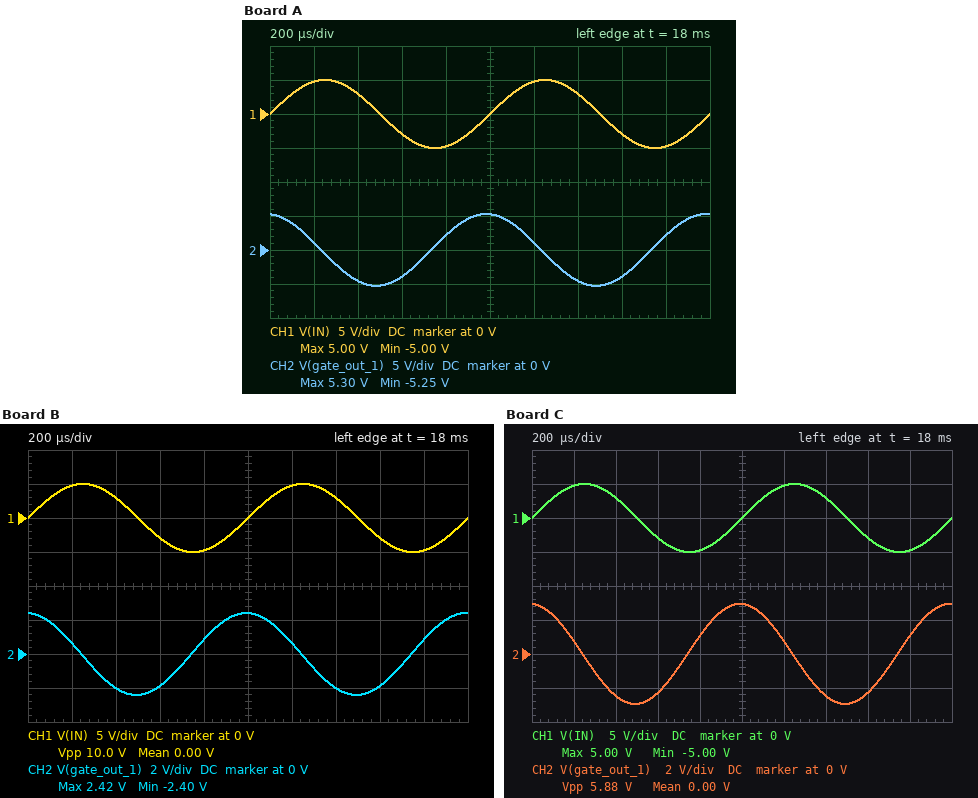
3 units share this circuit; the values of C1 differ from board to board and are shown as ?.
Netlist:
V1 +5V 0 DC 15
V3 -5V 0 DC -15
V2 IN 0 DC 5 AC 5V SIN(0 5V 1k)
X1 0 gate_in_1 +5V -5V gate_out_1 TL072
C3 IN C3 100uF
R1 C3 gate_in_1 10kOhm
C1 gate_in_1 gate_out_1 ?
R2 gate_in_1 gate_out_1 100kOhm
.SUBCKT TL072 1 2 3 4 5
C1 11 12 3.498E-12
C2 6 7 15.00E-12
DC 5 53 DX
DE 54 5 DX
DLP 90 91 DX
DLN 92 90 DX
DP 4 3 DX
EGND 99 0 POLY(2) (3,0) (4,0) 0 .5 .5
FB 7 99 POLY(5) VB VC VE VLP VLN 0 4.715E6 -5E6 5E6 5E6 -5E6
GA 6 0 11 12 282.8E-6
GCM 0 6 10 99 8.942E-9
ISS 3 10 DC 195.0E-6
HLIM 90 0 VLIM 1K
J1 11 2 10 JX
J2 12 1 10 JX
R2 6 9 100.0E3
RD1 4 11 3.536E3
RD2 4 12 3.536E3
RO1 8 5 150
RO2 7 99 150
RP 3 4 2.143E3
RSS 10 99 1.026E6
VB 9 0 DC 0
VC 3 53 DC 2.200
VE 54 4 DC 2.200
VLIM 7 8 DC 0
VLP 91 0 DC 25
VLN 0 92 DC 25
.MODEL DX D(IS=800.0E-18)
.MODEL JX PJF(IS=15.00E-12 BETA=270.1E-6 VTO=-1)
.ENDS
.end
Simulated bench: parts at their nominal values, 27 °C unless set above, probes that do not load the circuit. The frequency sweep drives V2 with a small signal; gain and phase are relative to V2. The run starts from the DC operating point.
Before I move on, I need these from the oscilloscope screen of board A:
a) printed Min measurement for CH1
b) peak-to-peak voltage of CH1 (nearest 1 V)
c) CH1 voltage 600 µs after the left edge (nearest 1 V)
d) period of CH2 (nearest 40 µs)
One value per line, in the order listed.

-5.00 V
10 V
-3 V
1.00 ms
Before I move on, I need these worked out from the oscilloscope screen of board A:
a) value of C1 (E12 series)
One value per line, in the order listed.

15 nF
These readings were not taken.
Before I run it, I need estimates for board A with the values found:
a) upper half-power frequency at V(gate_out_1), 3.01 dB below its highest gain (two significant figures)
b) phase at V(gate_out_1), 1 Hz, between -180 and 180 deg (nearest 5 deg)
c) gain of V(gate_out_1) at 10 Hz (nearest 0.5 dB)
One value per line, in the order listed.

110 Hz
-170 deg
20.0 dB
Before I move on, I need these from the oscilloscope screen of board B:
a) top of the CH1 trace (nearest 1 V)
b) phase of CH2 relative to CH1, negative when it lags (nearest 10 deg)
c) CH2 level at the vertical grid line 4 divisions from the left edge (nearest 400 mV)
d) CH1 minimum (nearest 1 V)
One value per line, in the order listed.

5 V
90 deg
800 mV
-5 V
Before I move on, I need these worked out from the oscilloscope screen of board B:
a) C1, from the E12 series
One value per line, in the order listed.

33 nF
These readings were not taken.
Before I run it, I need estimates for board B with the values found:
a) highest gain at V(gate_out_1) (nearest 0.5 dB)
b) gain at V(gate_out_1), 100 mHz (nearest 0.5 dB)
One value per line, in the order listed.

20.0 dB
14.5 dB
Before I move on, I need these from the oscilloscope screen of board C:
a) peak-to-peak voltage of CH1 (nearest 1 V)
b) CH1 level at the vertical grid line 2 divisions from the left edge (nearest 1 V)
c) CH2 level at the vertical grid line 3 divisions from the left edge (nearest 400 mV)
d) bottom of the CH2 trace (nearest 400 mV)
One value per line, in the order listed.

10 V
3 V
-2.4 V
-2.8 V
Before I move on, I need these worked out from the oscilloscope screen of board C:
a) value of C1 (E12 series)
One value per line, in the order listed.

27 nF
